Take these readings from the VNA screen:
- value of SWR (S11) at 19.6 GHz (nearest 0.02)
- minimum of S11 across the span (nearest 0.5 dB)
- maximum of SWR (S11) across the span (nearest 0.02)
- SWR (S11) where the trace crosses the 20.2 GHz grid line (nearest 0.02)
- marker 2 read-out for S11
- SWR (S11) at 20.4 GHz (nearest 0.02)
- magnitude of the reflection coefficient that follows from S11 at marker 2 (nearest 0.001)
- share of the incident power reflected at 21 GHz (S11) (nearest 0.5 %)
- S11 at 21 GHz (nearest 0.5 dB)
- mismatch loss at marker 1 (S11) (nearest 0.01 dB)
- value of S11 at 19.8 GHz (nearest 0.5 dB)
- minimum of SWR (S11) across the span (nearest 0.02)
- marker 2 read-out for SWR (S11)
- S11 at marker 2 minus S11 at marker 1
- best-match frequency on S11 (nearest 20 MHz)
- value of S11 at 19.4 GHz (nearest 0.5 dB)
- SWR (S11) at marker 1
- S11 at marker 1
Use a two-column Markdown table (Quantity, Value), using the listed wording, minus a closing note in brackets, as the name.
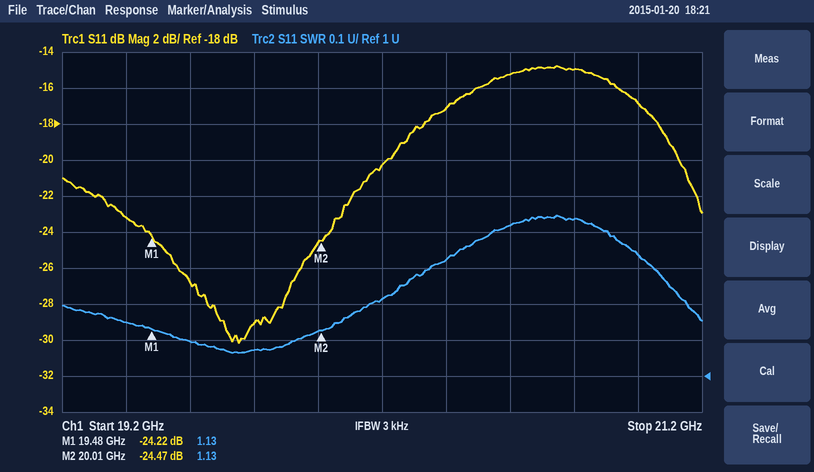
| Quantity | Value |
|---|---|
| value of SWR (S11) at 19.6 GHz | 1.10 |
| minimum of S11 across the span | -30.0 dB |
| maximum of SWR (S11) across the span | 1.44 |
| SWR (S11) where the trace crosses the 20.2 GHz grid line | 1.22 |
| marker 2 read-out for S11 | -24.47 dB |
| SWR (S11) at 20.4 GHz | 1.32 |
| magnitude of the reflection coefficient that follows from S11 at marker 2 | 0.060 |
| share of the incident power reflected at 21 GHz (S11) | 2.0 % |
| S11 at 21 GHz | -17.0 dB |
| mismatch loss at marker 1 (S11) | 0.02 dB |
| value of S11 at 19.8 GHz | -29.0 dB |
| minimum of SWR (S11) across the span | 1.06 |
| marker 2 read-out for SWR | 1.13 |
| S11 at marker 2 minus S11 at marker 1 | -0.25 dB |
| best-match frequency on S11 | 19.76 GHz |
| value of S11 at 19.4 GHz | -23.0 dB |
| SWR (S11) at marker 1 | 1.13 |
| S11 at marker 1 | -24.22 dB |
